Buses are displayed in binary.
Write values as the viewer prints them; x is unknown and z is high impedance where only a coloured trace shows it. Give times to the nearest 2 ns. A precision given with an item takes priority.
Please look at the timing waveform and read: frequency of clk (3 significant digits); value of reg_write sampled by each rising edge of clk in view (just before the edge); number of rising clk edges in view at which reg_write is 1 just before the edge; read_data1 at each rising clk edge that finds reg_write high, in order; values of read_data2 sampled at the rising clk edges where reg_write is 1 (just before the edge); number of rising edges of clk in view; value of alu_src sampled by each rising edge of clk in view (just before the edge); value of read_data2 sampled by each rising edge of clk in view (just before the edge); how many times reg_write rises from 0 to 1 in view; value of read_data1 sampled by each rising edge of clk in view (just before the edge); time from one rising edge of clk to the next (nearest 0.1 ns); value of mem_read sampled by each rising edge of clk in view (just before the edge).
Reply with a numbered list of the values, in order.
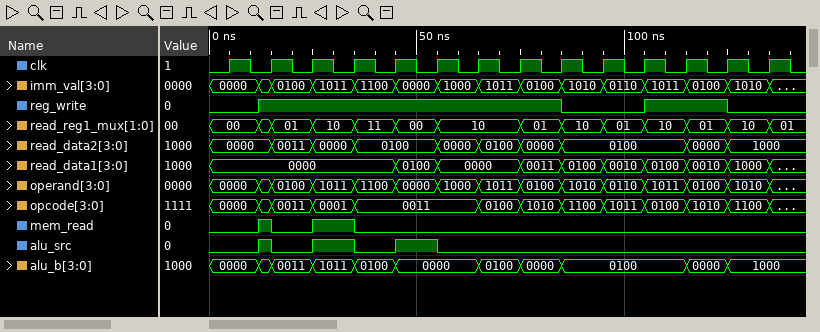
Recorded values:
1. 100 MHz
2. 0 1 1 1 1 1 1 1 1 0 0 1 1 0
3. 10
4. 0000, 0000, 0000, 0000, 0100, 0000, 0000, 0011, 0100, 0010
5. 0000, 0011, 0000, 0100, 0100, 0000, 0100, 0000, 0100, 0000
6. 14
7. 0 1 0 1 0 1 0 0 0 0 0 0 0 0
8. 0000, 0000, 0011, 0000, 0100, 0100, 0000, 0100, 0000, 0100, 0100, 0100, 0000, 1000
9. 2
10. 0000, 0000, 0000, 0000, 0000, 0100, 0000, 0000, 0011, 0100, 0010, 0100, 0010, 1000
11. 10 ns
12. 0 1 0 1 0 0 0 0 0 0 0 0 0 0
